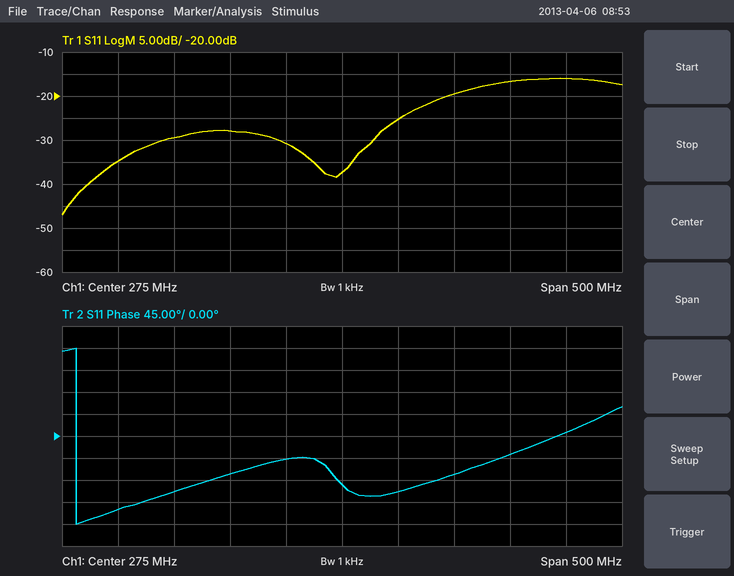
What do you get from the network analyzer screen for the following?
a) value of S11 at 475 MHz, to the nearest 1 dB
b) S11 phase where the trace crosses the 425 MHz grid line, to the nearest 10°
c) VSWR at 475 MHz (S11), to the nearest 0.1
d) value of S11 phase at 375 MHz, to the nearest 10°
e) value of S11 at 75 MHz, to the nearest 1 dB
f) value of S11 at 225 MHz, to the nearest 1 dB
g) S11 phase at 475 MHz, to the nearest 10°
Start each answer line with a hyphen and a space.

- -16 dB
- -40°
- 1.4
- -80°
- -35 dB
- -31 dB
- 10°
